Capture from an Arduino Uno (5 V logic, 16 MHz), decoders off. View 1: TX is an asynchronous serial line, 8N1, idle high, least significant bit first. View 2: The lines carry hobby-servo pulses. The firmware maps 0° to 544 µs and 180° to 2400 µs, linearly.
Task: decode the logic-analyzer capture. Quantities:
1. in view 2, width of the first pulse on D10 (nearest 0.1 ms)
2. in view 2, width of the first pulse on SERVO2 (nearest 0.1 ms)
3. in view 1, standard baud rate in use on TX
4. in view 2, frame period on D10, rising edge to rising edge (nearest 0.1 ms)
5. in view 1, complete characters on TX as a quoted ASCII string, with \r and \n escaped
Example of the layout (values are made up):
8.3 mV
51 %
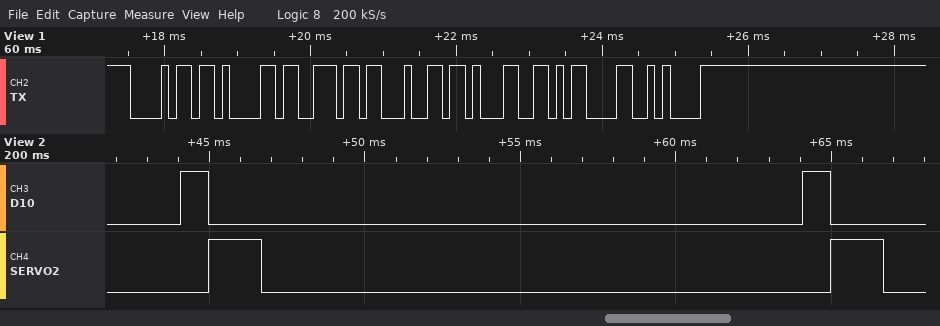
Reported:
0.9 ms
1.7 ms
9600 baud
20.0 ms
"hand1\r\n"
